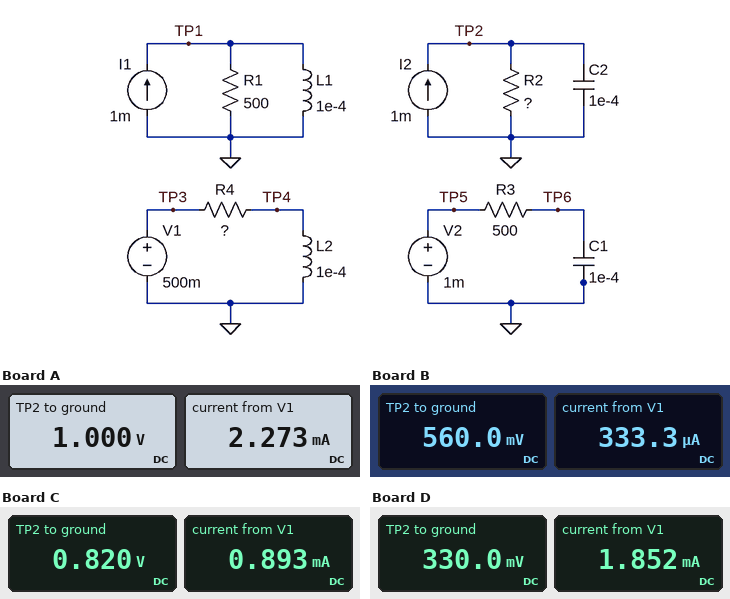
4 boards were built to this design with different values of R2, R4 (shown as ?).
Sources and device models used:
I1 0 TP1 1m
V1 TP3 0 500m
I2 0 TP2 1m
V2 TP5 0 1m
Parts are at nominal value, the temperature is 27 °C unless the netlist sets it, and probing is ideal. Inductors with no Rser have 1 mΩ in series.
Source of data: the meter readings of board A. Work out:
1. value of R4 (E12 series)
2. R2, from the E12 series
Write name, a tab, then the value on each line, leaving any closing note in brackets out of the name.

value of R4	220 Ω
R2, from the E12 series	1 kΩ
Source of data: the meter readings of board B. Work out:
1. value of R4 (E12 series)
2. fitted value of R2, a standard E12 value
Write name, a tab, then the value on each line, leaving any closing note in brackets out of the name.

value of R4	1.5 kΩ
fitted value of R2, a standard E12 value	560 Ω
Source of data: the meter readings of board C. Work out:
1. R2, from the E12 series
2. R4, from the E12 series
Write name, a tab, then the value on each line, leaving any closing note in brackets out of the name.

R2, from the E12 series	820 Ω
R4, from the E12 series	560 Ω
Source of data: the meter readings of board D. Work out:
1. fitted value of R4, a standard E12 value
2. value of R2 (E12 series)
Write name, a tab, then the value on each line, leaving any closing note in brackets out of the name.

fitted value of R4, a standard E12 value	270 Ω
value of R2	330 Ω
